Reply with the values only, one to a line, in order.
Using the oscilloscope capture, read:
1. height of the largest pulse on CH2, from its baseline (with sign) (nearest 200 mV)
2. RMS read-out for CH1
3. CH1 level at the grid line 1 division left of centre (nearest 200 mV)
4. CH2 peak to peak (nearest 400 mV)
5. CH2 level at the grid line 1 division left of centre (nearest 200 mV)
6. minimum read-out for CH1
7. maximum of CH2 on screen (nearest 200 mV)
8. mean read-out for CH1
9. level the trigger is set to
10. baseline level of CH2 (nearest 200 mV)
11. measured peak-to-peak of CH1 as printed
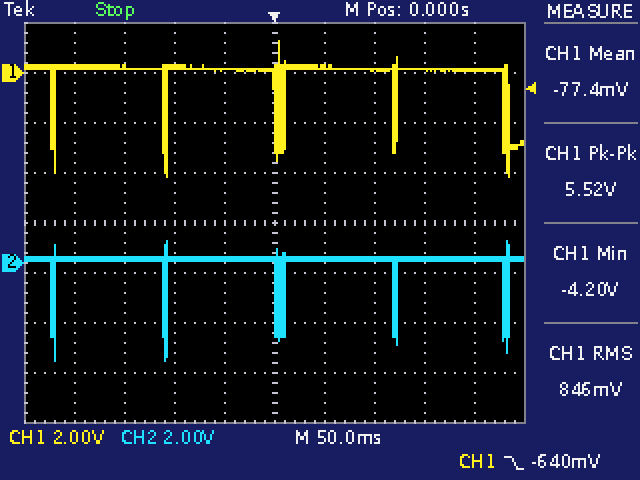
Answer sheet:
-4.0 V
846 mV
200 mV
4.8 V
200 mV
-4.20 V
800 mV
-77.4 mV
-640 mV
200 mV
5.52 V
